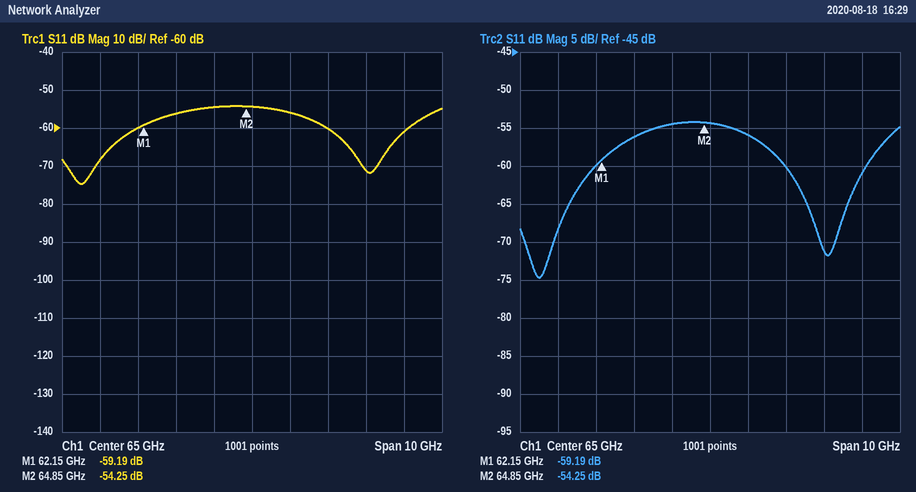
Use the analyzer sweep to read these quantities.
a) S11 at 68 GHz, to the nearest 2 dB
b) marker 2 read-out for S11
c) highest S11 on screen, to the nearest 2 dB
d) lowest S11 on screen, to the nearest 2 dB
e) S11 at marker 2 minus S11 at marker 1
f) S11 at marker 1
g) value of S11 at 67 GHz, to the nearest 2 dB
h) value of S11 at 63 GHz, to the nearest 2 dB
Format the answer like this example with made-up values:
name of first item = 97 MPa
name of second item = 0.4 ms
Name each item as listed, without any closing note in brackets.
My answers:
S11 at 68 GHz, to the nearest 2 dB = -72 dB
marker 2 read-out for S11 = -54.25 dB
highest S11 on screen, to the nearest 2 dB = -54 dB
lowest S11 on screen, to the nearest 2 dB = -74 dB
S11 at marker 2 minus S11 at marker 1 = 4.94 dB
S11 at marker 1 = -59.19 dB
value of S11 at 67 GHz, to the nearest 2 dB = -60 dB
value of S11 at 63 GHz, to the nearest 2 dB = -56 dB
